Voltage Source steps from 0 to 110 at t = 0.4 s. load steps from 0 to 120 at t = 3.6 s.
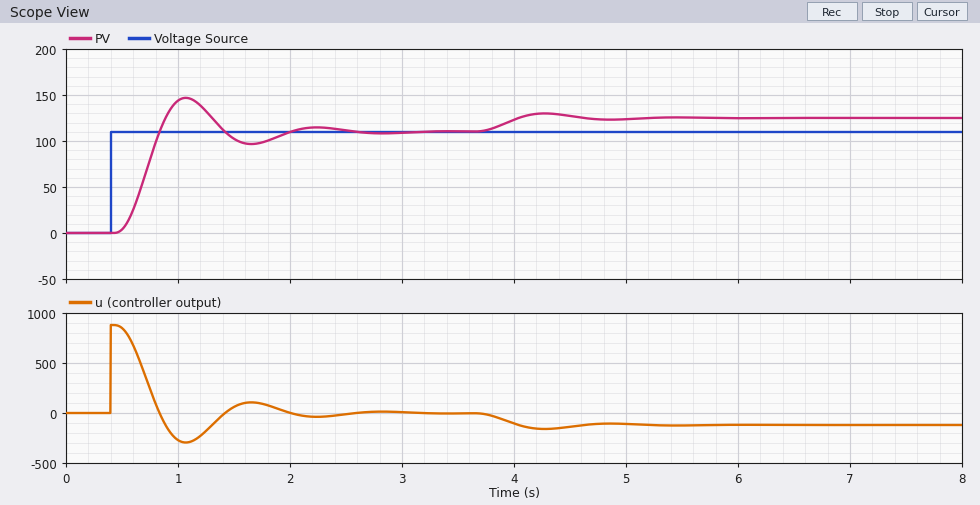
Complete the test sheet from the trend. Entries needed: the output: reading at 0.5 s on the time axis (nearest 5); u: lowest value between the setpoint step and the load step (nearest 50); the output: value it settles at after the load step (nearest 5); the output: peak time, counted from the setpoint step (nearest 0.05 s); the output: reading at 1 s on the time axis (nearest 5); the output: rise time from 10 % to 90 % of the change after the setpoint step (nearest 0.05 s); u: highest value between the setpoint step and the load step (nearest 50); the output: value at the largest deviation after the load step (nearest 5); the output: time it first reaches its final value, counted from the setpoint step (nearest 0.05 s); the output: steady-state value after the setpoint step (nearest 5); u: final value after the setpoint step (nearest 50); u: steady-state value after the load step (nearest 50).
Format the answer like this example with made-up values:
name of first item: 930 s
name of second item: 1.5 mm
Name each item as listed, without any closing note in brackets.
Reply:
the output: reading at 0.5 s on the time axis: 5
u: lowest value between the setpoint step and the load step: -300
the output: value it settles at after the load step: 125
the output: peak time, counted from the setpoint step: 0.65 s
the output: reading at 1 s on the time axis: 145
the output: rise time from 10 % to 90 % of the change after the setpoint step: 0.25 s
u: highest value between the setpoint step and the load step: 900
the output: value at the largest deviation after the load step: 130
the output: time it first reaches its final value, counted from the setpoint step: 0.45 s
the output: steady-state value after the setpoint step: 110
u: final value after the setpoint step: 0
u: steady-state value after the load step: -100
